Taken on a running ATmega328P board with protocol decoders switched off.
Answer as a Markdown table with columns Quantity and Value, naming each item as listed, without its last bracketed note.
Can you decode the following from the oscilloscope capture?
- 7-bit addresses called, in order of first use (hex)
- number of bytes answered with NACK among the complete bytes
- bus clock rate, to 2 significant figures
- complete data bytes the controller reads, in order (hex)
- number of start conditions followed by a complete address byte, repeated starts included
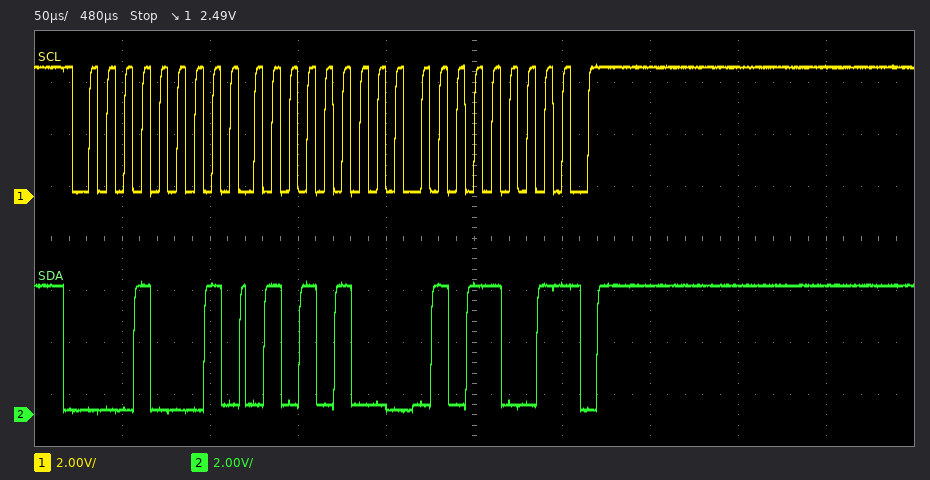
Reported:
| Quantity | Value |
|---|---|
| 7-bit addresses called, in order of first use | 0x08 |
| number of bytes answered with NACK among the complete bytes | 1 |
| bus clock rate, to 2 significant figures | 100 kHz |
| complete data bytes the controller reads, in order | 54 59 |
| number of start conditions followed by a complete address byte, repeated starts included | 1 |
